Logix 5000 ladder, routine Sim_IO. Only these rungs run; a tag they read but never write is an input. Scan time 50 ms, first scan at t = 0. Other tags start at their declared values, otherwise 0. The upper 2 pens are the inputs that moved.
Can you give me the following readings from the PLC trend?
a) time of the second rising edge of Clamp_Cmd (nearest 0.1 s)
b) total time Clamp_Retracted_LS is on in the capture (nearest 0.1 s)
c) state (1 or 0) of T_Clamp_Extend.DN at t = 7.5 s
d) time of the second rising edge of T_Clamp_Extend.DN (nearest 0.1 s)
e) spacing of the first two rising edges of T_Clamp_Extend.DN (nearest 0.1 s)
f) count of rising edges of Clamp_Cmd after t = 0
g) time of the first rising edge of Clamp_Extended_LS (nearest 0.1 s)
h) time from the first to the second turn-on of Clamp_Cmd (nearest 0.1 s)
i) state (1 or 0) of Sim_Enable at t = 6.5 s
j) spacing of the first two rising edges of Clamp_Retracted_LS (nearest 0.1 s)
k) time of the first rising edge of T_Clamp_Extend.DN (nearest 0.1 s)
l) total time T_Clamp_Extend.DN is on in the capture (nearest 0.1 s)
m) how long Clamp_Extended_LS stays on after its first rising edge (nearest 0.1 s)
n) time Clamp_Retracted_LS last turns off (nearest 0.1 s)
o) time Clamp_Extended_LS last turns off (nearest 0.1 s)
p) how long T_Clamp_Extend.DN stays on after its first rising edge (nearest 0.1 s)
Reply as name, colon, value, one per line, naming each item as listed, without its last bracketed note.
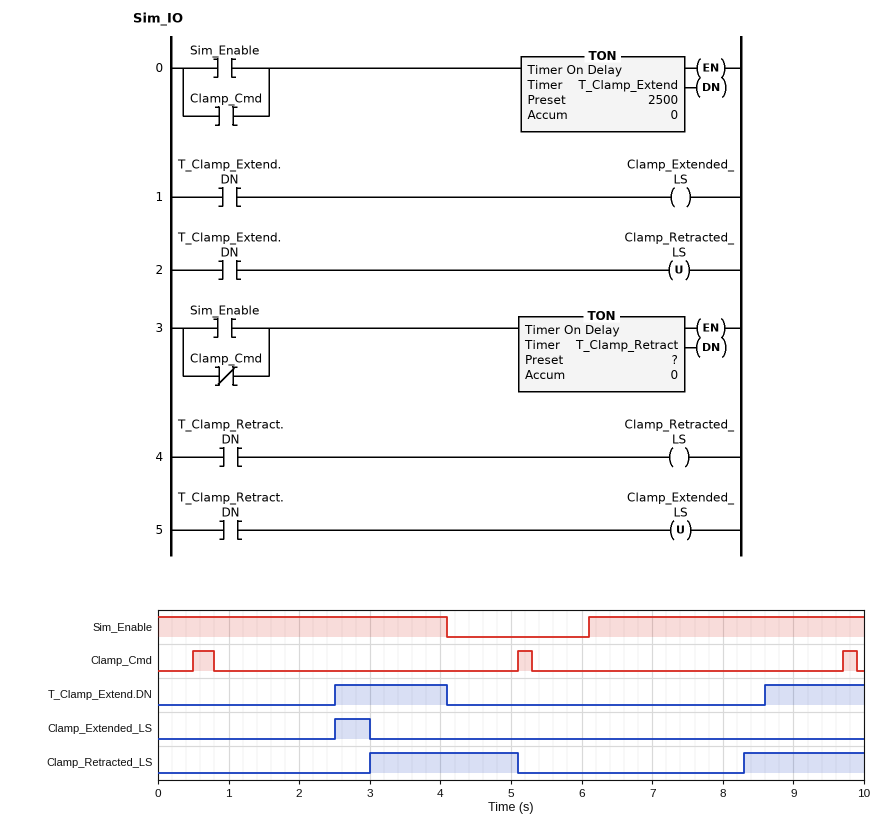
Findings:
time of the second rising edge of Clamp_Cmd: 5.1 s
total time Clamp_Retracted_LS is on in the capture: 3.8 s
state (1 or 0) of T_Clamp_Extend.DN at t = 7.5 s: 0
time of the second rising edge of T_Clamp_Extend.DN: 8.6 s
spacing of the first two rising edges of T_Clamp_Extend.DN: 6.1 s
count of rising edges of Clamp_Cmd after t = 0: 3
time of the first rising edge of Clamp_Extended_LS: 2.5 s
time from the first to the second turn-on of Clamp_Cmd: 4.6 s
state (1 or 0) of Sim_Enable at t = 6.5 s: 1
spacing of the first two rising edges of Clamp_Retracted_LS: 5.3 s
time of the first rising edge of T_Clamp_Extend.DN: 2.5 s
total time T_Clamp_Extend.DN is on in the capture: 3.0 s
how long Clamp_Extended_LS stays on after its first rising edge: 0.5 s
time Clamp_Retracted_LS last turns off: 5.1 s
time Clamp_Extended_LS last turns off: 3.0 s
how long T_Clamp_Extend.DN stays on after its first rising edge: 1.6 s
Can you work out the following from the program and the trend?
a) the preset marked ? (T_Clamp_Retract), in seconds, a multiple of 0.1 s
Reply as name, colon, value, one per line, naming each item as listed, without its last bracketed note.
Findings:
the preset marked ? (T_Clamp_Retract), in seconds, a multiple of 0.1 s: 3.0 s
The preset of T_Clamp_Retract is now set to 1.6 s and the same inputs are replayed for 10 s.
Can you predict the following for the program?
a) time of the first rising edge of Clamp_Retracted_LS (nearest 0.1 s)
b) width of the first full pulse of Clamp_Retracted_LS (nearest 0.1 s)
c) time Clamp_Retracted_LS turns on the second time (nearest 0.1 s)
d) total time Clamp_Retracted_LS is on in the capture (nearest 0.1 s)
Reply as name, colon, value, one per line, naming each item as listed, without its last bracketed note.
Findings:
time of the first rising edge of Clamp_Retracted_LS: 1.6 s
width of the first full pulse of Clamp_Retracted_LS: 3.5 s
time Clamp_Retracted_LS turns on the second time: 6.9 s
total time Clamp_Retracted_LS is on in the capture: 6.6 s
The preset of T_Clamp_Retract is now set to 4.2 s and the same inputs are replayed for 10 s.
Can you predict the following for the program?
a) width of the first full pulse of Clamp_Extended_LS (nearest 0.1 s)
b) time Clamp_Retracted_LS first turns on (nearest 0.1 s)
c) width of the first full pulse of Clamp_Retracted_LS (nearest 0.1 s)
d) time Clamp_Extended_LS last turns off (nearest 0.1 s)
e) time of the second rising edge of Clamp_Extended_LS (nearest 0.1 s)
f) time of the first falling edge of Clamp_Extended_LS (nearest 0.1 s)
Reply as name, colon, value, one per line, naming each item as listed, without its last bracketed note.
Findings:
width of the first full pulse of Clamp_Extended_LS: 1.6 s
time Clamp_Retracted_LS first turns on: 4.2 s
width of the first full pulse of Clamp_Retracted_LS: 0.9 s
time Clamp_Extended_LS last turns off: 9.5 s
time of the second rising edge of Clamp_Extended_LS: 8.6 s
time of the first falling edge of Clamp_Extended_LS: 4.1 s
